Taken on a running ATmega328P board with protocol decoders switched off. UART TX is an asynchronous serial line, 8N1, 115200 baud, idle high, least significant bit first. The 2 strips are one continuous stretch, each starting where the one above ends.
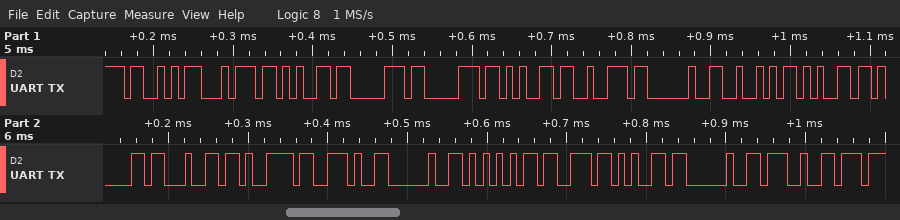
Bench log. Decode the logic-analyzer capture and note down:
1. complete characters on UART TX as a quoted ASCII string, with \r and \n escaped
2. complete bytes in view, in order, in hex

"Stepper Ready. Use '"
0x53 0x74 0x65 0x70 0x70 0x65 0x72 0x20 0x52 0x65 0x61 0x64 0x79 0x2E 0x20 0x55 0x73 0x65 0x20 0x27
